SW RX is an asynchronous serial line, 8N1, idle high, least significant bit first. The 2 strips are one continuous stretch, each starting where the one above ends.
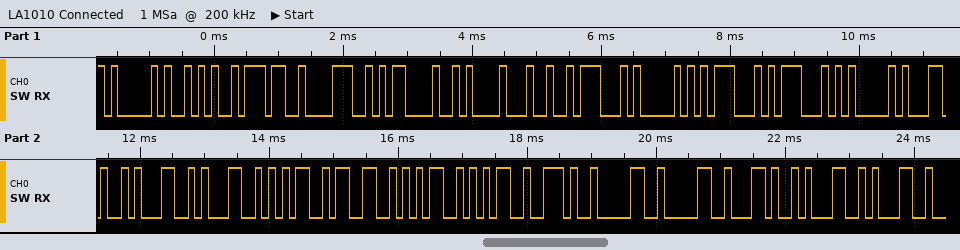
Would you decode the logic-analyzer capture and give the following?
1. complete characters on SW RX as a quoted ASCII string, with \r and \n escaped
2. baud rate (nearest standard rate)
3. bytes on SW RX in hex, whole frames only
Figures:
"A*78\r\n$GPGGA,115355.00,11"
9600 baud
41 2A 37 38 0D 0A 24 47 50 47 47 41 2C 31 31 35 33 35 35 2E 30 30 2C 31 31
